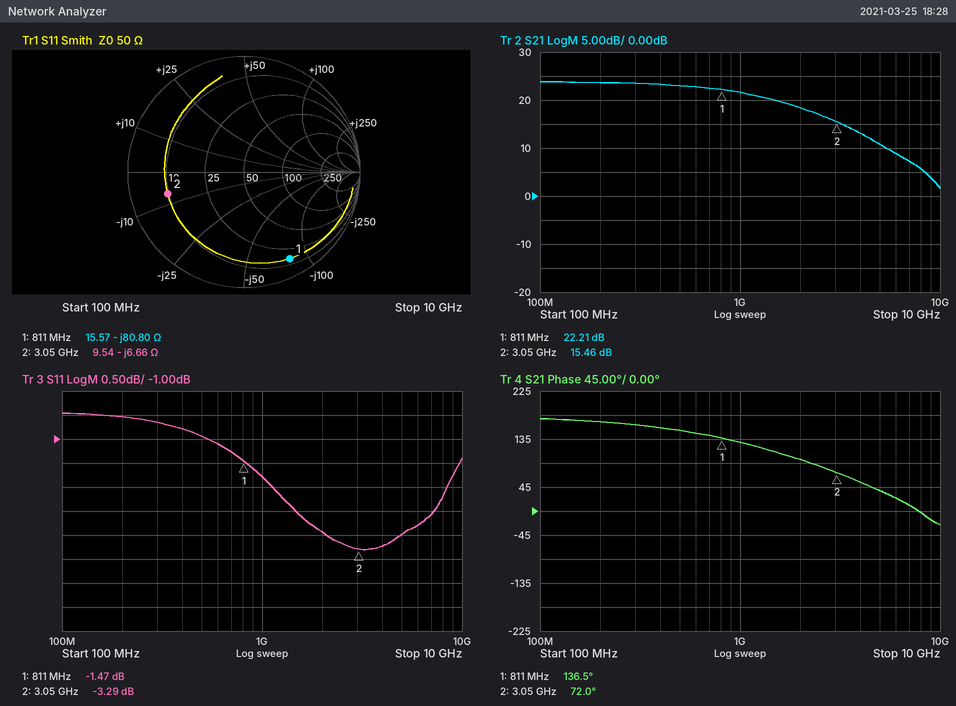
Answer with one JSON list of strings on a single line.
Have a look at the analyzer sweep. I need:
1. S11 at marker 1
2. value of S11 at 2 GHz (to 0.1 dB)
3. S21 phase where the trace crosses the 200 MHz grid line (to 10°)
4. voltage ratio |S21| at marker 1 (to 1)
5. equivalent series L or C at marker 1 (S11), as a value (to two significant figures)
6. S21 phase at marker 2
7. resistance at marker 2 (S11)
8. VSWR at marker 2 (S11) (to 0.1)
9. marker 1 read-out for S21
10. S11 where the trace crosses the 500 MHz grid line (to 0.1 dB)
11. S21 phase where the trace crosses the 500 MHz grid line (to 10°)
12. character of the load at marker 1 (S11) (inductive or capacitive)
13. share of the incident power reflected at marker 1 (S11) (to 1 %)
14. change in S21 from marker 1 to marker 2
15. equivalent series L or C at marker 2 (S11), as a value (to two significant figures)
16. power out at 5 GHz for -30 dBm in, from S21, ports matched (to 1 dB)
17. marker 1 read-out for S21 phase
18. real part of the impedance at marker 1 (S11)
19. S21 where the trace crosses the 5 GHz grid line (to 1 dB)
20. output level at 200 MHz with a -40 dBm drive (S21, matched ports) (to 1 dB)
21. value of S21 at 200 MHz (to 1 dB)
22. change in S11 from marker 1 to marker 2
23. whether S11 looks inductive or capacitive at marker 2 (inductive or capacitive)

["-1.47 dB", "-2.9 dB", "170°", "13", "2.4 pF", "72.0°", "9.54 Ω", "5.3", "22.21 dB", "-0.9 dB", "150°", "capacitive", "71 %", "-6.75 dB", "7.8 pF", "-19 dBm", "136.5°", "15.57 Ω", "11 dB", "-16 dBm", "24 dB", "-1.82 dB", "capacitive"]
